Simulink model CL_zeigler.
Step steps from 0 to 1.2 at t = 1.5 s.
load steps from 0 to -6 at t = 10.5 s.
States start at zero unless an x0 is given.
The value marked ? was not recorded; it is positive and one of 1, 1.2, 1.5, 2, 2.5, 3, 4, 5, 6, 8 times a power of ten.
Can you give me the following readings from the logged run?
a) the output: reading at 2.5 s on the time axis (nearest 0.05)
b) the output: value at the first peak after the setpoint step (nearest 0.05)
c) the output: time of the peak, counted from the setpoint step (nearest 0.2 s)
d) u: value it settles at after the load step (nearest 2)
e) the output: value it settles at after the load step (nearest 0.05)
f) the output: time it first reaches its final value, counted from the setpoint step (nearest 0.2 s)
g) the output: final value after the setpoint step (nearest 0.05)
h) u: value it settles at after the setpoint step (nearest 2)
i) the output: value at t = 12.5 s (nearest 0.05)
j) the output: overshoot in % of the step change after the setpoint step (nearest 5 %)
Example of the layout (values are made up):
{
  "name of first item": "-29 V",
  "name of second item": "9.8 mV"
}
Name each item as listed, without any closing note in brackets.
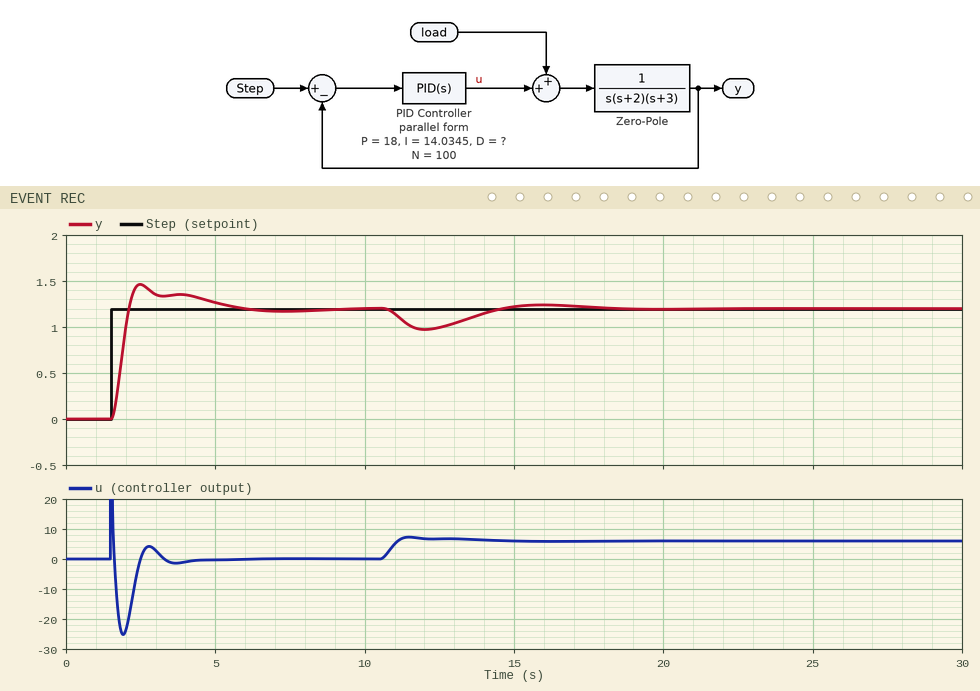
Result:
{
  "the output: reading at 2.5 s on the time axis": "1.45",
  "the output: value at the first peak after the setpoint step": "1.45",
  "the output: time of the peak, counted from the setpoint step": "1.0 s",
  "u: value it settles at after the load step": "6",
  "the output: value it settles at after the load step": "1.20",
  "the output: time it first reaches its final value, counted from the setpoint step": "0.6 s",
  "the output: final value after the setpoint step": "1.20",
  "u: value it settles at after the setpoint step": "0",
  "the output: value at t = 12.5 s": "1.00",
  "the output: overshoot in % of the step change after the setpoint step": "20 %"
}
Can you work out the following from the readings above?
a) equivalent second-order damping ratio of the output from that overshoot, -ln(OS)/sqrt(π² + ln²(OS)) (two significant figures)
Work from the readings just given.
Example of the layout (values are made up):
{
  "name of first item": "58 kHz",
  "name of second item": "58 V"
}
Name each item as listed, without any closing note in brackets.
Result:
{
  "equivalent second-order damping ratio of the output from that overshoot, -ln(OS)/sqrt(π² + ln²(OS))": "0.46"
}
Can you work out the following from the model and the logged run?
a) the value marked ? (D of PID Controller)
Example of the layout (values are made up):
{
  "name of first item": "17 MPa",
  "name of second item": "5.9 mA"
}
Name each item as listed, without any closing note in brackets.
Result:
{
  "the value marked ?": "15"
}
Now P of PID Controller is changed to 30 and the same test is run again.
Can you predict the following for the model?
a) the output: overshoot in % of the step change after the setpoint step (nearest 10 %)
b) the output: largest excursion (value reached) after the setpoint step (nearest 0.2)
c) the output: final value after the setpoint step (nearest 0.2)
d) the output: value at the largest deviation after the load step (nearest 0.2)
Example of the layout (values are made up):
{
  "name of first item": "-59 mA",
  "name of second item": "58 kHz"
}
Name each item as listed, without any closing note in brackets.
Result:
{
  "the output: overshoot in % of the step change after the setpoint step": "40 %",
  "the output: largest excursion (value reached) after the setpoint step": "1.6",
  "the output: final value after the setpoint step": "1.2",
  "the output: value at the largest deviation after the load step": "1.0"
}
